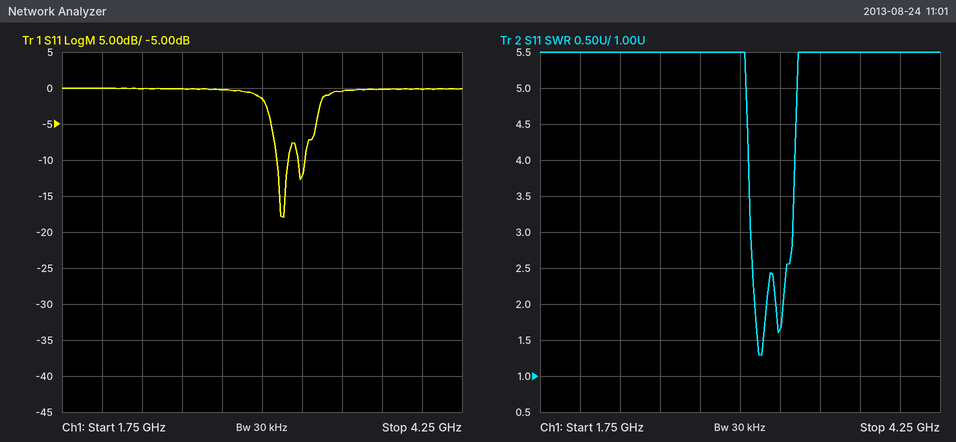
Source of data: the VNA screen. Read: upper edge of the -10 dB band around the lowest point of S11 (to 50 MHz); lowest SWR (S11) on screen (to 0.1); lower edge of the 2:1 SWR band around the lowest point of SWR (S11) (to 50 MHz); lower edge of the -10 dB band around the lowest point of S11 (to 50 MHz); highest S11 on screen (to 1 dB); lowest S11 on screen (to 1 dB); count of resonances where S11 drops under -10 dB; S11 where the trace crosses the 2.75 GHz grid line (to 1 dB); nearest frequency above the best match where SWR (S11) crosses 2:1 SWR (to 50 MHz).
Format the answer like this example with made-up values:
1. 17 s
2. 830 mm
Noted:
1. 3.15 GHz
2. 1.3
3. 3.10 GHz
4. 3.10 GHz
5. 0 dB
6. -18 dB
7. 2
8. 0 dB
9. 3.15 GHz
